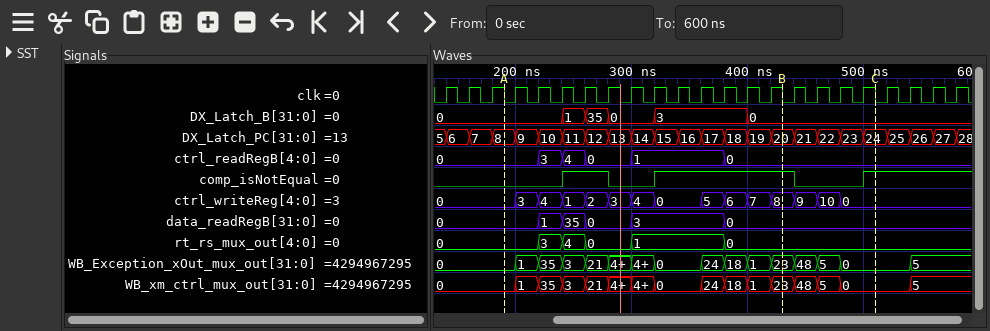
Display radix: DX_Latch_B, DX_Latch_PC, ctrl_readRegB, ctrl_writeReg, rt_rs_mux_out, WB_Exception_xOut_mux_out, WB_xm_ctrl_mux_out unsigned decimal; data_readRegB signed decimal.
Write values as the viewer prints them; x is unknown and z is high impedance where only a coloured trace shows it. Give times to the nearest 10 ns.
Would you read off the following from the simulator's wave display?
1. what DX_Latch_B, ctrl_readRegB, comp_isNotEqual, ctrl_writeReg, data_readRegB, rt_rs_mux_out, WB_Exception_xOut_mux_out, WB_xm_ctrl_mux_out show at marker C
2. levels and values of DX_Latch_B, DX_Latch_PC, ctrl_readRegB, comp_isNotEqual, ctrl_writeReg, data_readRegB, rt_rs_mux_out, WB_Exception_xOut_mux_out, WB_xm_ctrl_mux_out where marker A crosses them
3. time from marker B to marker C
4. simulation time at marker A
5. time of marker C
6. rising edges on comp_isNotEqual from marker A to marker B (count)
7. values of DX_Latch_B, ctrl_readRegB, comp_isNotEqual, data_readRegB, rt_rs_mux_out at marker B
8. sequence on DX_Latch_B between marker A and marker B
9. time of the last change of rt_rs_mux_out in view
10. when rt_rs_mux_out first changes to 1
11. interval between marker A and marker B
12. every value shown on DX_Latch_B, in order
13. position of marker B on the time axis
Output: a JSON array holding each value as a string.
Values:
["DX_Latch_B=0, ctrl_readRegB=0, comp_isNotEqual=1, ctrl_writeReg=0, data_readRegB=0, rt_rs_mux_out=0, WB_Exception_xOut_mux_out=0, WB_xm_ctrl_mux_out=0", "DX_Latch_B=0, DX_Latch_PC=8, ctrl_readRegB=0, comp_isNotEqual=0, ctrl_writeReg=0, data_readRegB=0, rt_rs_mux_out=0, WB_Exception_xOut_mux_out=0, WB_xm_ctrl_mux_out=0", "80 ns", "190 ns", "510 ns", "2", "DX_Latch_B=0, ctrl_readRegB=0, comp_isNotEqual=1, data_readRegB=0, rt_rs_mux_out=0", "0, 1, 35, 0, 3, 0", "380 ns", "300 ns", "240 ns", "0, 1, 35, 0, 3, 0", "430 ns"]
